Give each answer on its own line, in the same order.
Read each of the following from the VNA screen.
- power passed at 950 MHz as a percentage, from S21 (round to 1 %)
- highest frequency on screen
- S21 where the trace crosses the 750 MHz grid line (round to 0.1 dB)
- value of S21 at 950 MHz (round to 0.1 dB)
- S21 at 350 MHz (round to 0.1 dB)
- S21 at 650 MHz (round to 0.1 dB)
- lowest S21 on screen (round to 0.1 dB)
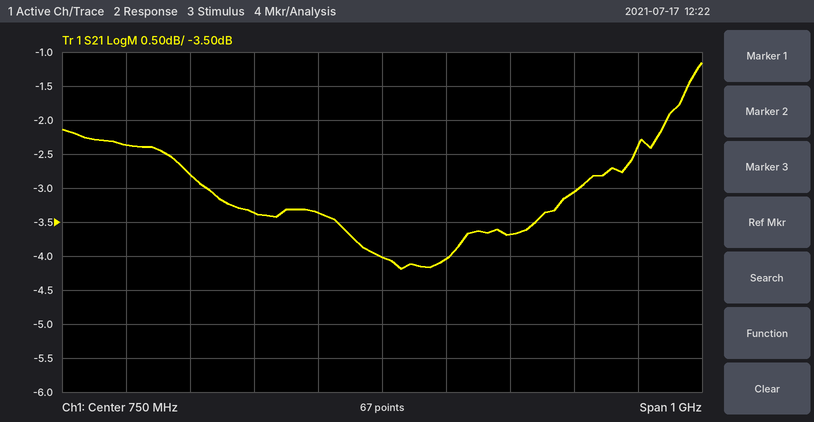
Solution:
43 %
1.25 GHz
-4.0 dB
-3.7 dB
-2.4 dB
-3.4 dB
-4.2 dB
